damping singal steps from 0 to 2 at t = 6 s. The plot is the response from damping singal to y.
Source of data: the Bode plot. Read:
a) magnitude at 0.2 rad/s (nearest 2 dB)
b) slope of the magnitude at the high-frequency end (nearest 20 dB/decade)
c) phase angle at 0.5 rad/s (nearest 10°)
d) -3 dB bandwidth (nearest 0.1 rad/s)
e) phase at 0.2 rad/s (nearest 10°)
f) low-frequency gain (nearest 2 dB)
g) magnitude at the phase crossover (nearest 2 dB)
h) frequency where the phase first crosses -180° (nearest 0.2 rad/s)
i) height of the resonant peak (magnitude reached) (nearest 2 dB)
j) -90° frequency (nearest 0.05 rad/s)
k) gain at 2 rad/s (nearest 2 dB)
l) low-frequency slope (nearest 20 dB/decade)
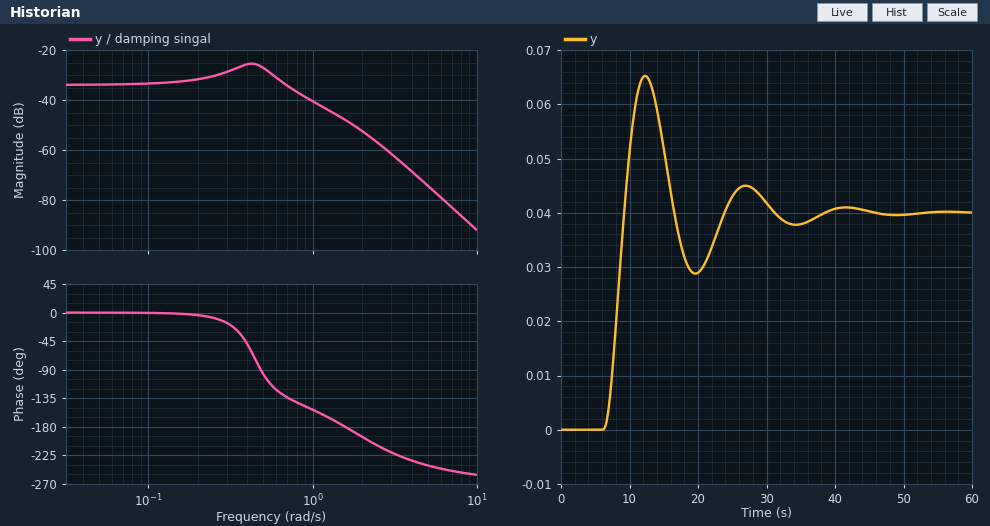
-32 dB
-60 dB/decade
-100°
0.8 rad/s
0°
-34 dB
-48 dB
1.6 rad/s
-26 dB
0.50 rad/s
-52 dB
0 dB/decade
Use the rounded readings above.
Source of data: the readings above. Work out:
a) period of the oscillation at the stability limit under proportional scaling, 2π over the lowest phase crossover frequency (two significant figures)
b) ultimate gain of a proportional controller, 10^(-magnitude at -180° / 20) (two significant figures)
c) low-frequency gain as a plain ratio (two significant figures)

3.9 s
250
0.020
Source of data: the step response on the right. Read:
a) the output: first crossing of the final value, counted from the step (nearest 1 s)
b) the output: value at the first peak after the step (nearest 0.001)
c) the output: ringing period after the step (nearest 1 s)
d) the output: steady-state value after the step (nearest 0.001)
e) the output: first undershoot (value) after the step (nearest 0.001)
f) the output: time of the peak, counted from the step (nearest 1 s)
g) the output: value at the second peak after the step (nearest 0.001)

3 s
0.065
15 s
0.040
0.029
6 s
0.045
